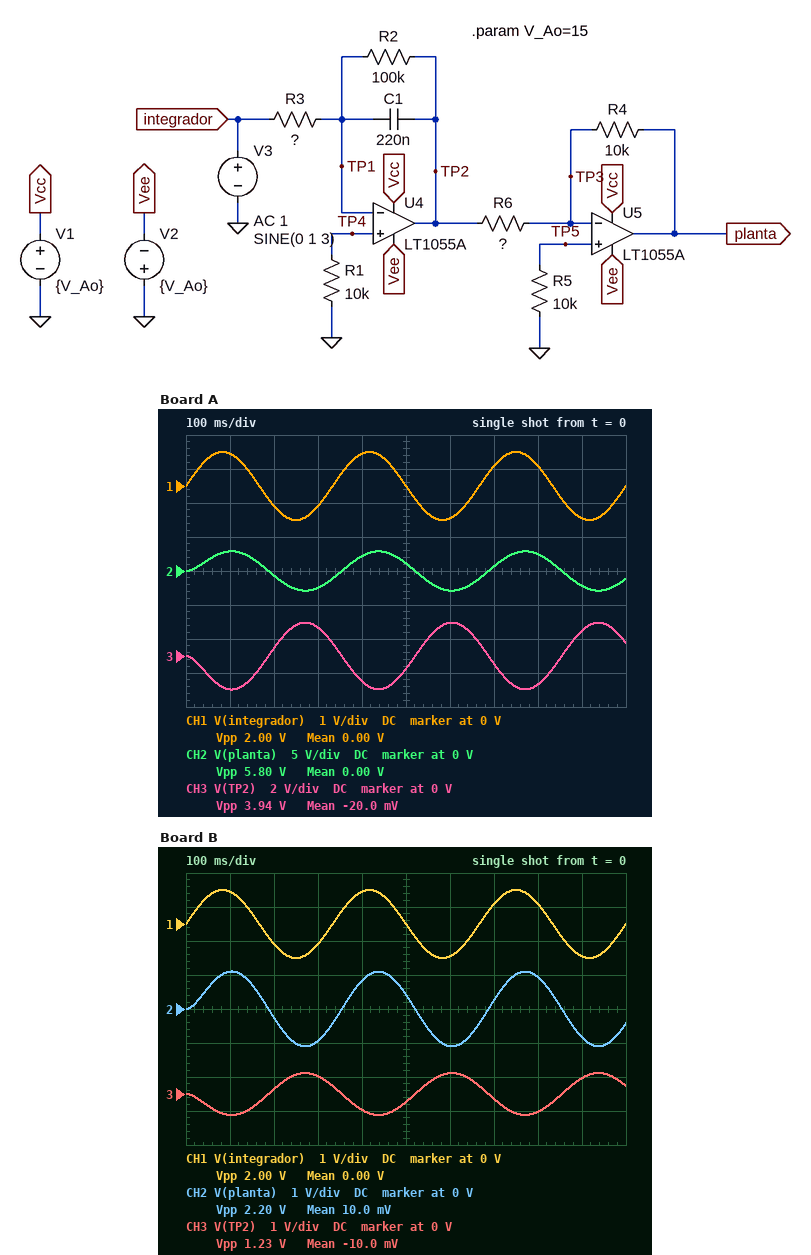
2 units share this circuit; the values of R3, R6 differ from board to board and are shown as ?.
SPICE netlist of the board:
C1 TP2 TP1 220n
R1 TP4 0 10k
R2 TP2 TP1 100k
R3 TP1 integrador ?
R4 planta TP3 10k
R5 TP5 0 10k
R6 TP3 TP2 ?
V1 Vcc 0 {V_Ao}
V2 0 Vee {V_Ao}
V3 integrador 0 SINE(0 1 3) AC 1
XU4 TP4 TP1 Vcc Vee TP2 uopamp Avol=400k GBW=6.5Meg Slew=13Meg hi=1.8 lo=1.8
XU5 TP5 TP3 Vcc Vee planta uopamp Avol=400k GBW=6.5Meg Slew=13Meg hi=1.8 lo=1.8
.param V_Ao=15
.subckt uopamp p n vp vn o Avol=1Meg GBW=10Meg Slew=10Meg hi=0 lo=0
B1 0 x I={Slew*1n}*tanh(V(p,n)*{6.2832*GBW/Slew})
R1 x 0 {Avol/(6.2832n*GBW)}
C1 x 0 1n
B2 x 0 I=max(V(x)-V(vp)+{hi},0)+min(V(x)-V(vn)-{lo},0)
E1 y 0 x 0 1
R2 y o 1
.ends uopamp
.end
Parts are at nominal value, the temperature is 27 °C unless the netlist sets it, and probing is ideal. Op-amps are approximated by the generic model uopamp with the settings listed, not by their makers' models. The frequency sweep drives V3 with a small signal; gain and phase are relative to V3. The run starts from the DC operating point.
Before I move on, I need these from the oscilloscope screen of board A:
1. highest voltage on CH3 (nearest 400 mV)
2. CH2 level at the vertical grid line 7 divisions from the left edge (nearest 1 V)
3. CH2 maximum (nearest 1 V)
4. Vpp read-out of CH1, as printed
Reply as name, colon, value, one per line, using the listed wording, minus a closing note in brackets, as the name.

highest voltage on CH3: 2.0 V
CH2 level at the vertical grid line 7 divisions from the left edge: 1 V
CH2 maximum: 3 V
Vpp read-out of CH1, as printed: 2.00 V
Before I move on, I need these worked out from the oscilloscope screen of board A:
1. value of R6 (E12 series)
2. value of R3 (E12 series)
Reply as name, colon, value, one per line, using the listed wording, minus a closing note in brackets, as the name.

value of R6: 6.8 kΩ
value of R3: 47 kΩ
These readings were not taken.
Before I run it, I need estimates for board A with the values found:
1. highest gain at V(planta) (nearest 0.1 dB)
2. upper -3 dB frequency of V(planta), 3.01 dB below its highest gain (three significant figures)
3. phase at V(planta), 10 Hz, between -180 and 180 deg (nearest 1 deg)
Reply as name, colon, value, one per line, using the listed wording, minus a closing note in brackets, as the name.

highest gain at V(planta): 9.9 dB
upper -3 dB frequency of V(planta), 3.01 dB below its highest gain: 7.23 Hz
phase at V(planta), 10 Hz, between -180 and 180 deg: -54 deg
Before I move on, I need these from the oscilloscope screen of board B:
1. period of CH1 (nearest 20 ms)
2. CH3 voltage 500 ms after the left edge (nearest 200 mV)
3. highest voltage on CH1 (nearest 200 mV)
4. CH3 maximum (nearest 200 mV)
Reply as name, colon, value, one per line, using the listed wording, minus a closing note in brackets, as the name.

period of CH1: 340 ms
CH3 voltage 500 ms after the left edge: -200 mV
highest voltage on CH1: 1.0 V
CH3 maximum: 600 mV
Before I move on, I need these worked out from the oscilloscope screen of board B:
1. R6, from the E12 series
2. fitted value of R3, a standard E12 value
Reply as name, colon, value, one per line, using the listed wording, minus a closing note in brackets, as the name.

R6, from the E12 series: 5.6 kΩ
fitted value of R3, a standard E12 value: 150 kΩ
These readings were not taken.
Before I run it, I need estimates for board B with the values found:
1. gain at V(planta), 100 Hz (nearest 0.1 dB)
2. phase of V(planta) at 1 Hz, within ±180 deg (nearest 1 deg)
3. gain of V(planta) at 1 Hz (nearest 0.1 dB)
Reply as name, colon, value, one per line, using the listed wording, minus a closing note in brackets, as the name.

gain at V(planta), 100 Hz: -21.3 dB
phase of V(planta) at 1 Hz, within ±180 deg: -8 deg
gain of V(planta) at 1 Hz: 1.4 dB
